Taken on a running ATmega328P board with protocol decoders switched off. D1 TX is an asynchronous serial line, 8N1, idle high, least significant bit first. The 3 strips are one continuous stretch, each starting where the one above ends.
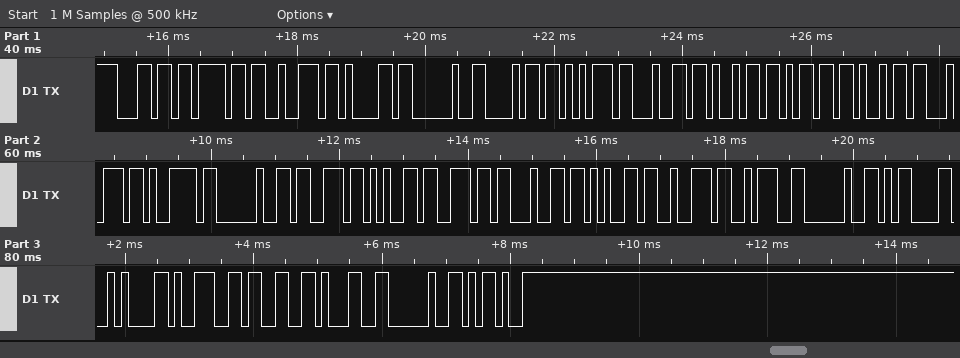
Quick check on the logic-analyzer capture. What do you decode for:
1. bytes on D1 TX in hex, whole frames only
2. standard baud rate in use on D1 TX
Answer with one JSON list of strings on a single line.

["6C 6F 72 61 20 68 75 64 69 6D 69 74 79 20 73 65 6E 64 65 72 3A 20 0D 0A 39 33 31 20 2D", "9600 baud"]
